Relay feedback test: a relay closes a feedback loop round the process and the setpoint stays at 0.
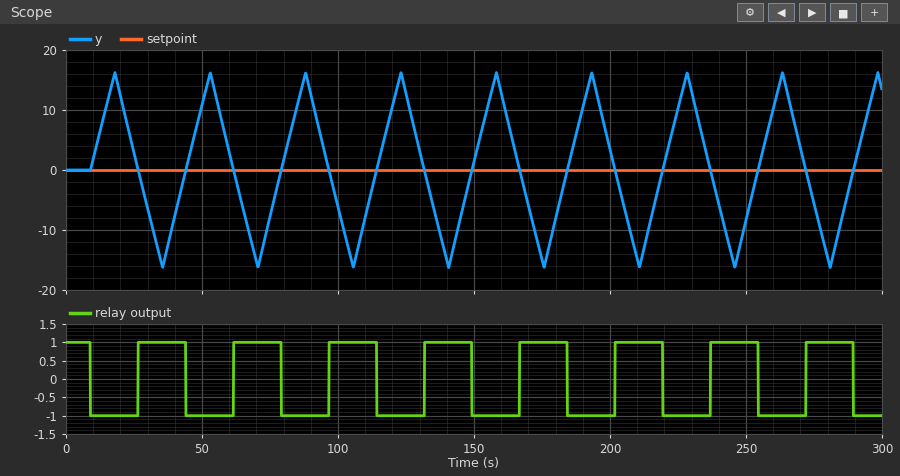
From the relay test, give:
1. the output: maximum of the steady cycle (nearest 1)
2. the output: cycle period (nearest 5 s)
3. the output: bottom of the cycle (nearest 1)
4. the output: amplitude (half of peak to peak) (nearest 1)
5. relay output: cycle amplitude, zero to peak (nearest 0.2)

16
35 s
-16
16
1.0
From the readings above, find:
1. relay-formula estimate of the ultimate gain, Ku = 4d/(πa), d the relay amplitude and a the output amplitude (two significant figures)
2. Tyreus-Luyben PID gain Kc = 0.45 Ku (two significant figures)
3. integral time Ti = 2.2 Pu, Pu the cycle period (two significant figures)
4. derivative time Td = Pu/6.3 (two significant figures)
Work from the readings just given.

0.080
0.036
77 s
5.6 s
